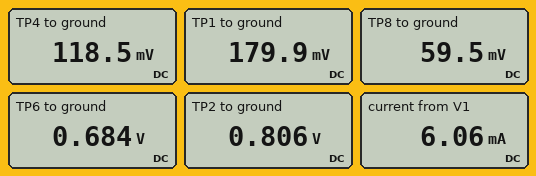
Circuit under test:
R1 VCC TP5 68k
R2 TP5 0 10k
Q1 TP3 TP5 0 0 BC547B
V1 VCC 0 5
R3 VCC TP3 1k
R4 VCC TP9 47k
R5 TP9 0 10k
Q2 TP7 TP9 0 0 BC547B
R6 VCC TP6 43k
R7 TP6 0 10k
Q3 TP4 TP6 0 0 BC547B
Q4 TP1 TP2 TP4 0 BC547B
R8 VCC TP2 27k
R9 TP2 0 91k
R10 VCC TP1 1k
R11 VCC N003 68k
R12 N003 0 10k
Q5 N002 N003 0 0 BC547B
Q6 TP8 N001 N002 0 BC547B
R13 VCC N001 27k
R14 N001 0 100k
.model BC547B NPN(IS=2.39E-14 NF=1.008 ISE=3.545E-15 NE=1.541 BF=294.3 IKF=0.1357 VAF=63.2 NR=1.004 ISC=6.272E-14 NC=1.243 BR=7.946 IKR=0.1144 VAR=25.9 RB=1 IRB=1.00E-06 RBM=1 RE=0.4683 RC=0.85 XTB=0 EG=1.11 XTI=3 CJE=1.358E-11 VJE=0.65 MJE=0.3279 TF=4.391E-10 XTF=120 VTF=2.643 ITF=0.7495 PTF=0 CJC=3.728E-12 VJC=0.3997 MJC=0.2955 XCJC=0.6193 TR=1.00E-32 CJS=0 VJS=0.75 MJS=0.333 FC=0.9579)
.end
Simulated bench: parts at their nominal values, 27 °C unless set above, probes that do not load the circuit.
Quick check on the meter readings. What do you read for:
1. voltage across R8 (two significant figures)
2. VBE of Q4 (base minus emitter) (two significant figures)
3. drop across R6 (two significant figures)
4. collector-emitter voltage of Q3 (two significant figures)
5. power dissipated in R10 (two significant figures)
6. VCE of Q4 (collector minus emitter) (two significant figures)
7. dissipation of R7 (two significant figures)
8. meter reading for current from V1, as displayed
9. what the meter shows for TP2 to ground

4.2 V
690 mV
4.3 V
120 mV
23 mW
61 mV
47 µW
6.06 mA
0.806 V
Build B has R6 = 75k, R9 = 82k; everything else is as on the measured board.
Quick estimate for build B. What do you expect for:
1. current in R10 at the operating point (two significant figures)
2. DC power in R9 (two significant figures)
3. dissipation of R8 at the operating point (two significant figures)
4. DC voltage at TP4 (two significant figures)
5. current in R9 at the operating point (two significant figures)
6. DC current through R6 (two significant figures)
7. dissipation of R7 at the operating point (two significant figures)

130 µA
170 µW
58 µW
3.2 V
46 µA
59 µA
34 µW
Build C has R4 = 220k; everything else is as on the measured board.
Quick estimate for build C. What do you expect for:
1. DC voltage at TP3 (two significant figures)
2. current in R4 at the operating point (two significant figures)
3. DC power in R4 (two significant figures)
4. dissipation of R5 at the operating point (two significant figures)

4.4 V
22 µA
100 µW
4.7 µW
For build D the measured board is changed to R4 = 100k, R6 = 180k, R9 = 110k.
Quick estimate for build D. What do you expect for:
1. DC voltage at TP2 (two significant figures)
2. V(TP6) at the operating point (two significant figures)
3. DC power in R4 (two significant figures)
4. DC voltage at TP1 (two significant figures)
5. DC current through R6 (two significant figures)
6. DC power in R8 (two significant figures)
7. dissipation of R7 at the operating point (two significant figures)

4.0 V
260 mV
210 µW
5.0 V
26 µA
36 µW
6.9 µW
